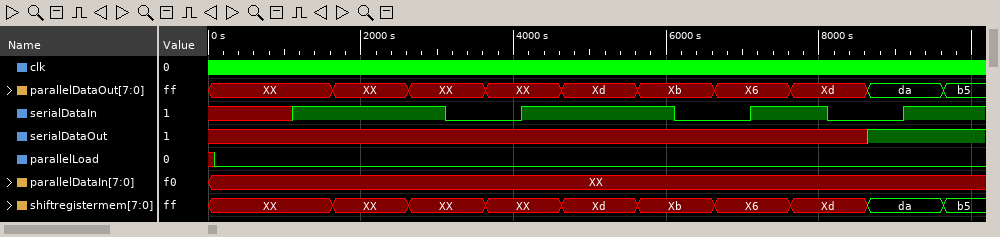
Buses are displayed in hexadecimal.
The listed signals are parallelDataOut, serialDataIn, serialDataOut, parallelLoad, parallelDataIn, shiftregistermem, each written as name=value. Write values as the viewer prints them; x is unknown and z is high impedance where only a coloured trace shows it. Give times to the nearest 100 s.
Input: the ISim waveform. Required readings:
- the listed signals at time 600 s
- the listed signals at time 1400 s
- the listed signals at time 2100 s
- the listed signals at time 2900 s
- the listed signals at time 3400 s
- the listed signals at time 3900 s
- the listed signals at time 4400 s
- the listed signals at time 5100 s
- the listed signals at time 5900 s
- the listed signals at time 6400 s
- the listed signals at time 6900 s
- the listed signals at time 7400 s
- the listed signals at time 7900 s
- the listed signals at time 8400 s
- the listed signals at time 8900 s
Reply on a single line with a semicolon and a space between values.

parallelDataOut=XX, serialDataIn=x, serialDataOut=x, parallelLoad=0, parallelDataIn=XX, shiftregistermem=XX; parallelDataOut=XX, serialDataIn=1, serialDataOut=x, parallelLoad=0, parallelDataIn=XX, shiftregistermem=XX; parallelDataOut=XX, serialDataIn=1, serialDataOut=x, parallelLoad=0, parallelDataIn=XX, shiftregistermem=XX; parallelDataOut=XX, serialDataIn=1, serialDataOut=x, parallelLoad=0, parallelDataIn=XX, shiftregistermem=XX; parallelDataOut=XX, serialDataIn=0, serialDataOut=x, parallelLoad=0, parallelDataIn=XX, shiftregistermem=XX; parallelDataOut=XX, serialDataIn=0, serialDataOut=x, parallelLoad=0, parallelDataIn=XX, shiftregistermem=XX; parallelDataOut=XX, serialDataIn=1, serialDataOut=x, parallelLoad=0, parallelDataIn=XX, shiftregistermem=XX; parallelDataOut=Xd, serialDataIn=1, serialDataOut=x, parallelLoad=0, parallelDataIn=XX, shiftregistermem=Xd; parallelDataOut=Xb, serialDataIn=1, serialDataOut=x, parallelLoad=0, parallelDataIn=XX, shiftregistermem=Xb; parallelDataOut=Xb, serialDataIn=0, serialDataOut=x, parallelLoad=0, parallelDataIn=XX, shiftregistermem=Xb; parallelDataOut=X6, serialDataIn=0, serialDataOut=x, parallelLoad=0, parallelDataIn=XX, shiftregistermem=X6; parallelDataOut=X6, serialDataIn=1, serialDataOut=x, parallelLoad=0, parallelDataIn=XX, shiftregistermem=X6; parallelDataOut=Xd, serialDataIn=1, serialDataOut=x, parallelLoad=0, parallelDataIn=XX, shiftregistermem=Xd; parallelDataOut=Xd, serialDataIn=0, serialDataOut=x, parallelLoad=0, parallelDataIn=XX, shiftregistermem=Xd; parallelDataOut=da, serialDataIn=0, serialDataOut=1, parallelLoad=0, parallelDataIn=XX, shiftregistermem=da
